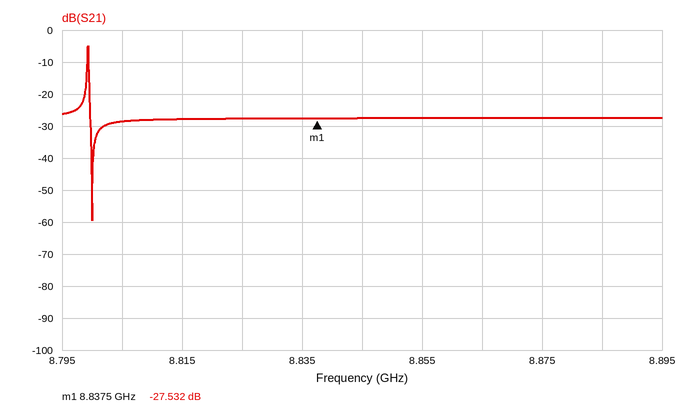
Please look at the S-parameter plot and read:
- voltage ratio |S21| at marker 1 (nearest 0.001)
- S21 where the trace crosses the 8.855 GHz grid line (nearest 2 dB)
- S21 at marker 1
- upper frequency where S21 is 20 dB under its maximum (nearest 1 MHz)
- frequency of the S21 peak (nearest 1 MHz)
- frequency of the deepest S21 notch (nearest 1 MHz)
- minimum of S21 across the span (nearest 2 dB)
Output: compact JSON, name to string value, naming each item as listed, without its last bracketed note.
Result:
{"voltage ratio |S21| at marker 1": "0.042", "S21 where the trace crosses the 8.855 GHz grid line": "-28 dB", "S21 at marker 1": "-27.532 dB", "upper frequency where S21 is 20 dB under its maximum": "8.800 GHz", "frequency of the S21 peak": "8.799 GHz", "frequency of the deepest S21 notch": "8.800 GHz", "minimum of S21 across the span": "-60 dB"}
